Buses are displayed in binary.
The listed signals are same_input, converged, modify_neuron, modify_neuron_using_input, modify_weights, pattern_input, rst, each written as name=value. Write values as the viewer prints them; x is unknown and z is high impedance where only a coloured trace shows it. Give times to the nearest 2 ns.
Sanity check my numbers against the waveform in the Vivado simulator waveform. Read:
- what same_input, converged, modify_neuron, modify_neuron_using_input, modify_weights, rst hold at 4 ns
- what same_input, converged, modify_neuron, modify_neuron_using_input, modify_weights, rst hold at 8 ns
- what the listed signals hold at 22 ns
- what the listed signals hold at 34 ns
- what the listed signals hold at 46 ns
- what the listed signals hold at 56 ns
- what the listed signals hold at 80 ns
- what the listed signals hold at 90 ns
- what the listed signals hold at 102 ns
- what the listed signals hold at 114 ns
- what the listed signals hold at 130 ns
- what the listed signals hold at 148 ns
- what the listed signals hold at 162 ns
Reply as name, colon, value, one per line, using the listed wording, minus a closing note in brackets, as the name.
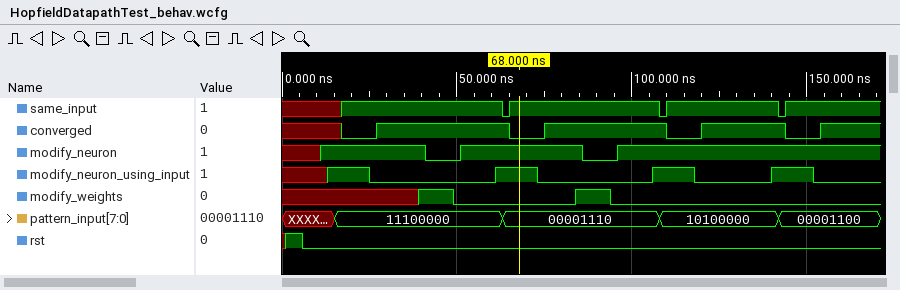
what same_input, converged, modify_neuron, modify_neuron_using_input, modify_weights, rst hold at 4 ns: same_input=x, converged=x, modify_neuron=x, modify_neuron_using_input=x, modify_weights=x, rst=1
what same_input, converged, modify_neuron, modify_neuron_using_input, modify_weights, rst hold at 8 ns: same_input=x, converged=x, modify_neuron=x, modify_neuron_using_input=x, modify_weights=x, rst=0
what the listed signals hold at 22 ns: same_input=1, converged=0, modify_neuron=1, modify_neuron_using_input=1, modify_weights=x, pattern_input=11100000, rst=0
what the listed signals hold at 34 ns: same_input=1, converged=1, modify_neuron=1, modify_neuron_using_input=0, modify_weights=x, pattern_input=11100000, rst=0
what the listed signals hold at 46 ns: same_input=1, converged=1, modify_neuron=0, modify_neuron_using_input=0, modify_weights=1, pattern_input=11100000, rst=0
what the listed signals hold at 56 ns: same_input=1, converged=1, modify_neuron=1, modify_neuron_using_input=0, modify_weights=0, pattern_input=11100000, rst=0
what the listed signals hold at 80 ns: same_input=1, converged=1, modify_neuron=1, modify_neuron_using_input=0, modify_weights=0, pattern_input=00001110, rst=0
what the listed signals hold at 90 ns: same_input=1, converged=1, modify_neuron=0, modify_neuron_using_input=0, modify_weights=1, pattern_input=00001110, rst=0
what the listed signals hold at 102 ns: same_input=1, converged=1, modify_neuron=1, modify_neuron_using_input=0, modify_weights=0, pattern_input=00001110, rst=0
what the listed signals hold at 114 ns: same_input=1, converged=0, modify_neuron=1, modify_neuron_using_input=1, modify_weights=0, pattern_input=10100000, rst=0
what the listed signals hold at 130 ns: same_input=1, converged=1, modify_neuron=1, modify_neuron_using_input=0, modify_weights=0, pattern_input=10100000, rst=0
what the listed signals hold at 148 ns: same_input=1, converged=0, modify_neuron=1, modify_neuron_using_input=1, modify_weights=0, pattern_input=00001100, rst=0
what the listed signals hold at 162 ns: same_input=1, converged=1, modify_neuron=1, modify_neuron_using_input=0, modify_weights=0, pattern_input=00001100, rst=0
